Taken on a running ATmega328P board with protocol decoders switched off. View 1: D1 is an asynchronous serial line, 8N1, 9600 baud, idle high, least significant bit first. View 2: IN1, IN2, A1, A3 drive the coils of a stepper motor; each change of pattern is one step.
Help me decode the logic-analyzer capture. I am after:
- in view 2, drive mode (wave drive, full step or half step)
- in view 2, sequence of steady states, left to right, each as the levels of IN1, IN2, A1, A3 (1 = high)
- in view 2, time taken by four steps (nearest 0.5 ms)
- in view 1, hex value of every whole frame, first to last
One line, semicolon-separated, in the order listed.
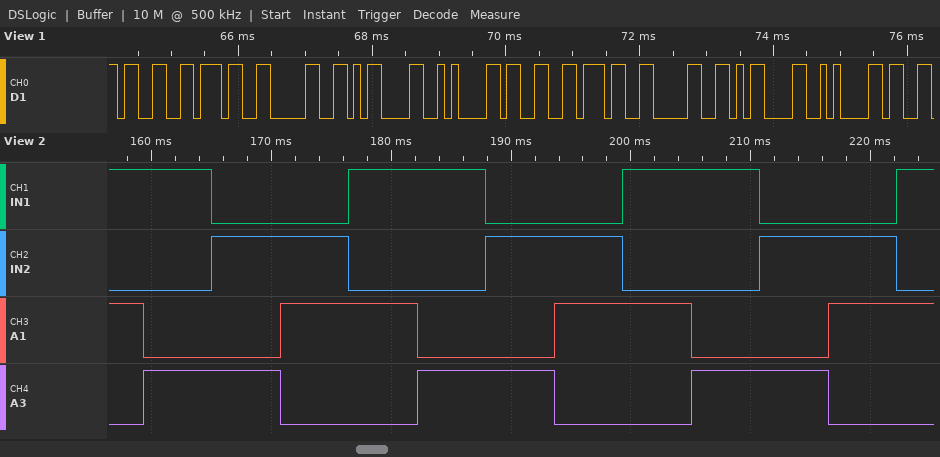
full step; 1010 1001 0101 0110 1010 1001 0101 0110 1010 1001 0101 0110 1010; 23.0 ms; 33 37 30 0D 0A 33 37 30 0D 0A
